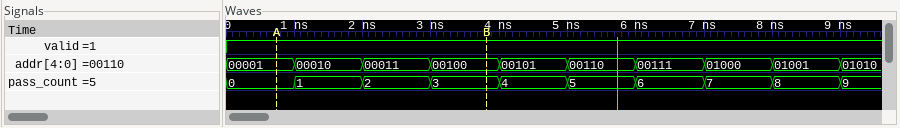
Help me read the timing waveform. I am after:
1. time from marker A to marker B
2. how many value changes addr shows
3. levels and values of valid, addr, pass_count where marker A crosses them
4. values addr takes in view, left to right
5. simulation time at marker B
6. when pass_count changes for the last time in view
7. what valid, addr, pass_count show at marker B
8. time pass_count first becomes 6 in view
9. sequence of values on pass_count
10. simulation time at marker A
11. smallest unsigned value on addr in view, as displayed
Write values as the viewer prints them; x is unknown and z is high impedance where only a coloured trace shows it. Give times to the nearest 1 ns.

3 ns
9
valid=1, addr=00001, pass_count=0
00001, 00010, 00011, 00100, 00101, 00110, 00111, 01000, 01001, 01010
4 ns
9 ns
valid=1, addr=00100, pass_count=3
6 ns
0, 1, 2, 3, 4, 5, 6, 7, 8, 9
1 ns
00001
